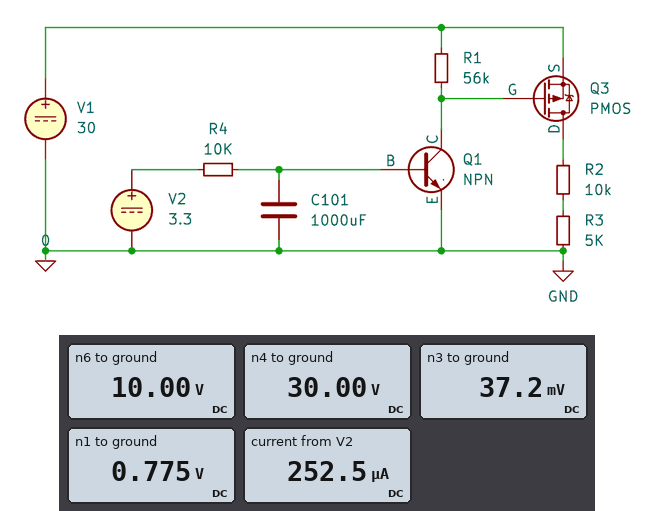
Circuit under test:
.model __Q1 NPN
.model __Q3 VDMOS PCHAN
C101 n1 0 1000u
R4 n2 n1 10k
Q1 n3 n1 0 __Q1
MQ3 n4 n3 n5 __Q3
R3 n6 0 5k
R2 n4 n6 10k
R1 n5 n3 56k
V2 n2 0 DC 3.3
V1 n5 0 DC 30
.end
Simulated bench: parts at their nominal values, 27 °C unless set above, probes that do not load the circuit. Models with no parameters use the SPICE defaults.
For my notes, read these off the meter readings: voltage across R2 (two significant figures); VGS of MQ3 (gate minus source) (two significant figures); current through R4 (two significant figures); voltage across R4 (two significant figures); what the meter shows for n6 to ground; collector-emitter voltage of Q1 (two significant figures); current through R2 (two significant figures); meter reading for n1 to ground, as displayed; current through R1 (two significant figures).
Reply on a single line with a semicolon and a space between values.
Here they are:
20 V; -30 V; 250 µA; 2.5 V; 10.00 V; 37 mV; 2.0 mA; 0.775 V; 540 µA
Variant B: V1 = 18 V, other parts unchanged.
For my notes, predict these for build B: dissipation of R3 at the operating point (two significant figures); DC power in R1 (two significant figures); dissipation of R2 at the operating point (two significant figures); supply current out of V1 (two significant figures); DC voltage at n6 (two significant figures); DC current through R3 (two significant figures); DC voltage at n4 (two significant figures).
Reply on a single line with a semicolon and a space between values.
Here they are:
7.2 mW; 5.8 mW; 14 mW; 1.5 mA; 6.0 V; 1.2 mA; 18 V
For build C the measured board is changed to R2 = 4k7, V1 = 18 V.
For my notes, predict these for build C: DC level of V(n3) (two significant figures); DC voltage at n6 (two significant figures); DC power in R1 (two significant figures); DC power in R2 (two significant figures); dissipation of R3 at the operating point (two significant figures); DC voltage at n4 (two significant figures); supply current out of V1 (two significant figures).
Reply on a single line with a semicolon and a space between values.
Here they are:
31 mV; 9.3 V; 5.8 mW; 16 mW; 17 mW; 18 V; 2.2 mA
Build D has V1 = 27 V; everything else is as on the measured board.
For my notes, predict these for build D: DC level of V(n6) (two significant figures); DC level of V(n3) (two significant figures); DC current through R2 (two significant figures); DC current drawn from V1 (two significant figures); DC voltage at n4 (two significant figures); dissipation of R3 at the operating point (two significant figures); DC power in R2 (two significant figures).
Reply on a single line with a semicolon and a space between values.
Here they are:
9.0 V; 36 mV; 1.8 mA; 2.3 mA; 27 V; 16 mW; 32 mW
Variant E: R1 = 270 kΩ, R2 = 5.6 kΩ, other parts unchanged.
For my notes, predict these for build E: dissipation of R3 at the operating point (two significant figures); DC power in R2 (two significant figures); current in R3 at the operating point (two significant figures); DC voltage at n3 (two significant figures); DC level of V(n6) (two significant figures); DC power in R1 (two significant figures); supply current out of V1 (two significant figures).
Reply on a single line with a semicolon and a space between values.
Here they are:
40 mW; 45 mW; 2.8 mA; 23 mV; 14 V; 3.3 mW; 2.9 mA
